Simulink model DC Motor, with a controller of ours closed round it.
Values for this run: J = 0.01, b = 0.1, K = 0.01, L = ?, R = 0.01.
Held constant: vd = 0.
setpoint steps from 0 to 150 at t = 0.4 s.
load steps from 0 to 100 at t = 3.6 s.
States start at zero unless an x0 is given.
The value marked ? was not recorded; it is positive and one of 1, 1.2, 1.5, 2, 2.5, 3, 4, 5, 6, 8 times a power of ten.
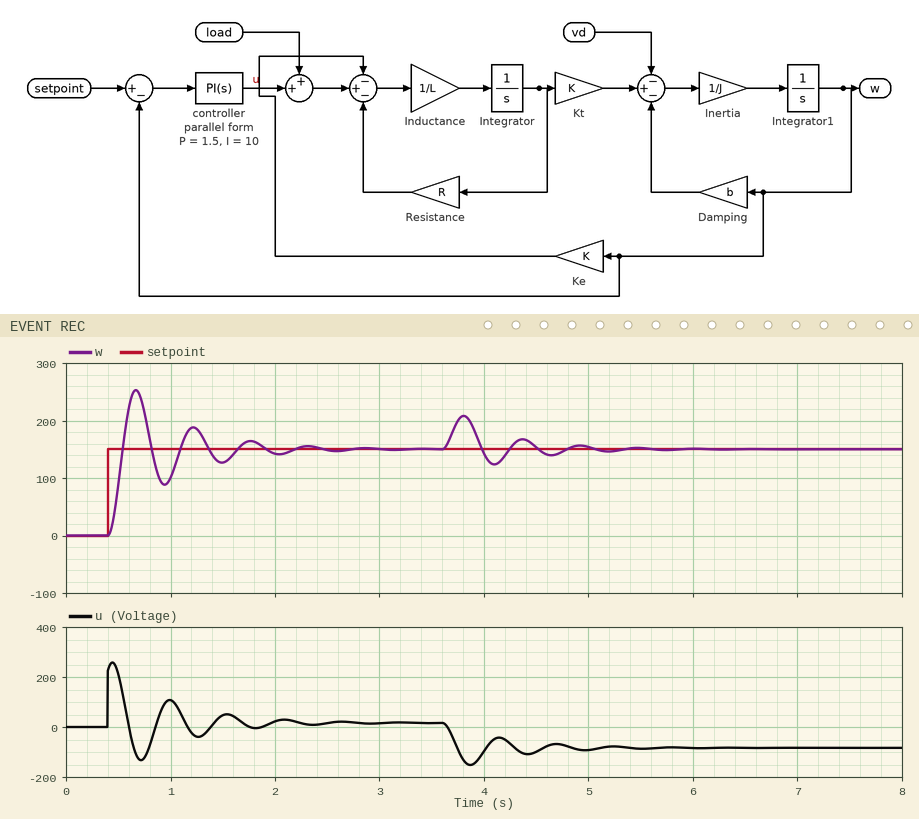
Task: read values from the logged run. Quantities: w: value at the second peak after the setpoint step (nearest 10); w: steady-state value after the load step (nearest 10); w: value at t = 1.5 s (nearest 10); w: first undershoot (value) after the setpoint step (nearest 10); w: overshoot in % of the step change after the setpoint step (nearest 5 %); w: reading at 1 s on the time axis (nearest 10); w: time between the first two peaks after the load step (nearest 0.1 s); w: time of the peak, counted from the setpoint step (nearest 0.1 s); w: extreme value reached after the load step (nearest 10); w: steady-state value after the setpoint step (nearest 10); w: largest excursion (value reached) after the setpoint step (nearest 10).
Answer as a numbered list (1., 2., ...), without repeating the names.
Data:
1. 190
2. 150
3. 130
4. 90
5. 70 %
6. 100
7. 0.6 s
8. 0.3 s
9. 210
10. 150
11. 250
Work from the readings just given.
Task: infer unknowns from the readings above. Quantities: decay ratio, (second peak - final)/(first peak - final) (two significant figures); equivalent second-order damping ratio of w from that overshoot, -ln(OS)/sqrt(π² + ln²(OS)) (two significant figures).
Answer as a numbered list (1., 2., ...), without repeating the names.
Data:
1. 0.40
2. 0.11
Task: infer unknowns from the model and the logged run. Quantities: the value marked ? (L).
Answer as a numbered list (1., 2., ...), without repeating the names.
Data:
1. 0.01
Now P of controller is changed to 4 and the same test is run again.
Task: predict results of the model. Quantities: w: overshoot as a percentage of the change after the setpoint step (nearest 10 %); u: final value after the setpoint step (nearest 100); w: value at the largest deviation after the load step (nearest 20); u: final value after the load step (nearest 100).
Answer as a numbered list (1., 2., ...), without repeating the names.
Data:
1. 50 %
2. 0
3. 180
4. -100
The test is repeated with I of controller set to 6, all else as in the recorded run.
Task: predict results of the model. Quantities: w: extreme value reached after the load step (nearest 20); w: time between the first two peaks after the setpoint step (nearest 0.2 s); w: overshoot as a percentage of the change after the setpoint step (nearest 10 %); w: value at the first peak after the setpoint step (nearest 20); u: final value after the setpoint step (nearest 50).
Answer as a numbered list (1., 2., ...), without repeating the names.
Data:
1. 220
2. 0.6 s
3. 50 %
4. 220
5. 0
